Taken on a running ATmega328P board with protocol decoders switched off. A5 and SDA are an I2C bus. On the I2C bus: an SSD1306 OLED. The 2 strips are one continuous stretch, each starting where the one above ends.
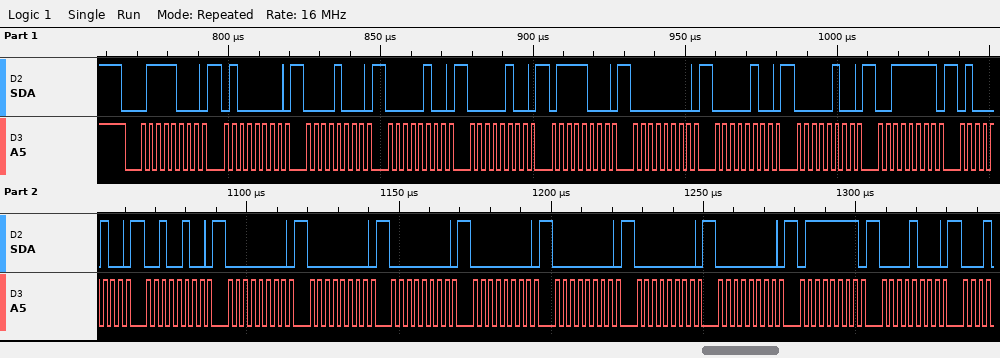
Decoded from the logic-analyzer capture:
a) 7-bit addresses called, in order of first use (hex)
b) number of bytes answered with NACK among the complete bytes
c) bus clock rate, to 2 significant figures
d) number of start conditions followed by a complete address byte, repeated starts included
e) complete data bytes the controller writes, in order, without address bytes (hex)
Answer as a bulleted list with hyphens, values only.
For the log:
- 0x3C
- 0
- 400 kHz
- 1
- 40 08 04 04 78 00 04 04 3F 44 24 00 00 00 00 00 00 00 7F 08
